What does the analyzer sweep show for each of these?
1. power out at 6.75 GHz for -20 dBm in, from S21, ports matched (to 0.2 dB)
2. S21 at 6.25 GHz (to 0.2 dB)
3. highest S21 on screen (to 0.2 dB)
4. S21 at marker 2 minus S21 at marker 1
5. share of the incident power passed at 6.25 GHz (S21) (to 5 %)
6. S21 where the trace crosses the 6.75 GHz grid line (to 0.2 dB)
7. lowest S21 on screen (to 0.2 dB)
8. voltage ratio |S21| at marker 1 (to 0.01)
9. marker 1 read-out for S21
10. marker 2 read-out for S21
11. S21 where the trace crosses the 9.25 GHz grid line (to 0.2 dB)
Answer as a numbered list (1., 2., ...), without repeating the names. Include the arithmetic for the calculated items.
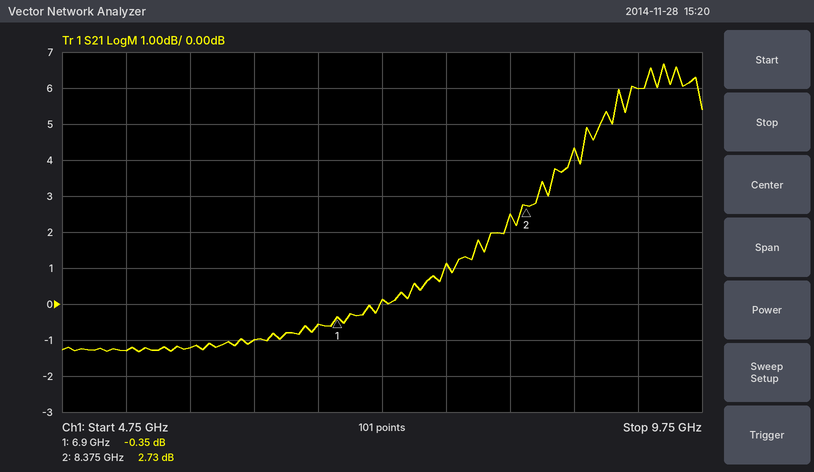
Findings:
1. -20 dBm + (-0.6 dB) = -20.6 dBm
2. -1.0 dB
3. 6.6 dB
4. 2.73 − (-0.35) = 3.08 dB
5. 10^(-1/10) ≈ 79.4 %, so 80 % to the nearest 5 %
6. -0.6 dB
7. -1.4 dB
8. 10^(-0.35/20) ≈ 0.96
9. -0.35 dB
10. 2.73 dB
11. 6.0 dB
